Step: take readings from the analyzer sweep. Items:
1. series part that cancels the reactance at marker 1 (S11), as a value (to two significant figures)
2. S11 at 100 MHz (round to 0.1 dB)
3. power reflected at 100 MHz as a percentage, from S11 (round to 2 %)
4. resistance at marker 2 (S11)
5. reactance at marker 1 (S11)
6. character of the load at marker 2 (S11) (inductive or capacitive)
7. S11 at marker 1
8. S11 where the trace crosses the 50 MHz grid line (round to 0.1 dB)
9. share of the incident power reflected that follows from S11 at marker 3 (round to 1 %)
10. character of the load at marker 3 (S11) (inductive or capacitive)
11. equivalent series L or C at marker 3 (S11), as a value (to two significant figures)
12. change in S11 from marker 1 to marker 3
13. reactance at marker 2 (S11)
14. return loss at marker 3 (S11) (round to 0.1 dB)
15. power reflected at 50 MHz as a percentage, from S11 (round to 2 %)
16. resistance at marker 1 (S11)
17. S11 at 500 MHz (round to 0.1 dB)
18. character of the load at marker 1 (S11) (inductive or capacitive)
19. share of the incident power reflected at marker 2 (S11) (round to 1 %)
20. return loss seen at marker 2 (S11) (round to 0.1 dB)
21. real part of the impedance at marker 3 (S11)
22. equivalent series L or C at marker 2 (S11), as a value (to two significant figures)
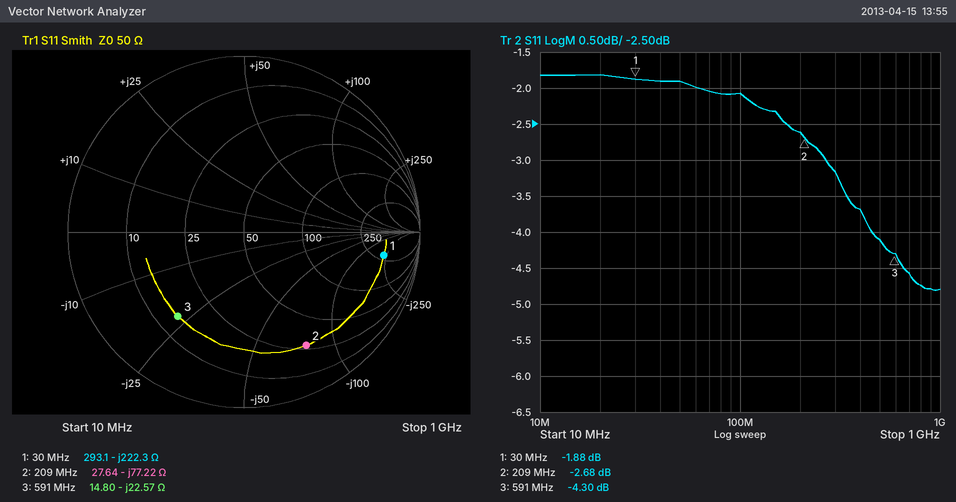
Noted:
1.2 µH
-2.1 dB
62 %
27.64 Ω
-222.3 Ω
capacitive
-1.88 dB
-1.9 dB
37 %
capacitive
12 pF
-2.42 dB
-77.22 Ω
4.3 dB
64 %
293.1 Ω
-4.1 dB
capacitive
54 %
2.7 dB
14.80 Ω
9.9 pF
